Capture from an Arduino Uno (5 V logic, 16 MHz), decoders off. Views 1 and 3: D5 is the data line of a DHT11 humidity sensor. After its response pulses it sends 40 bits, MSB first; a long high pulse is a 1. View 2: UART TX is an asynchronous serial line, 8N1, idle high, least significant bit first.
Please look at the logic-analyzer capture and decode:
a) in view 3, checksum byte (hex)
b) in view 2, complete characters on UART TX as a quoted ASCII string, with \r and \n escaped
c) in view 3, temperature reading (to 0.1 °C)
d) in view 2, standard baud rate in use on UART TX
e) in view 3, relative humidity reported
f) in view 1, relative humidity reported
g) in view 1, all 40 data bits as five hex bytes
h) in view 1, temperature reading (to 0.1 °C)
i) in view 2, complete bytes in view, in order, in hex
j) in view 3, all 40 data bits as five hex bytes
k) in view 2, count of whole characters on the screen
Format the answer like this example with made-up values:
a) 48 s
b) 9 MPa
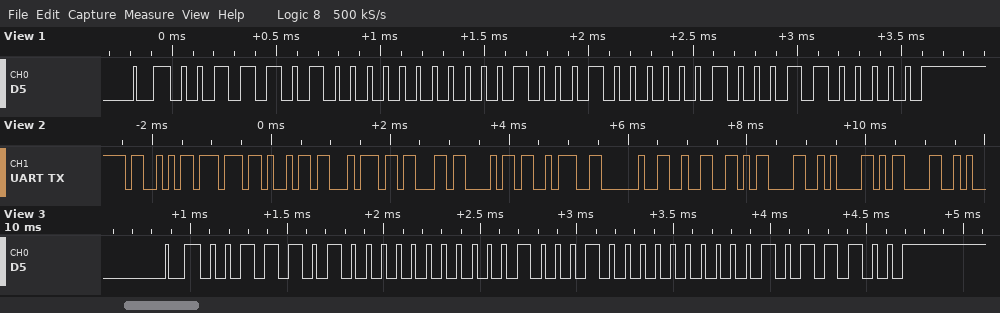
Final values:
a) 0x5C
b) "Switch: 2\r\n\r"
c) 34.0 °C
d) 9600 baud
e) 58 %
f) 58 %
g) 3A 00 22 04 60
h) 34.4 °C
i) 53 77 69 74 63 68 3A 20 32 0D 0A 0D
j) 3A 00 22 00 5C
k) 12
